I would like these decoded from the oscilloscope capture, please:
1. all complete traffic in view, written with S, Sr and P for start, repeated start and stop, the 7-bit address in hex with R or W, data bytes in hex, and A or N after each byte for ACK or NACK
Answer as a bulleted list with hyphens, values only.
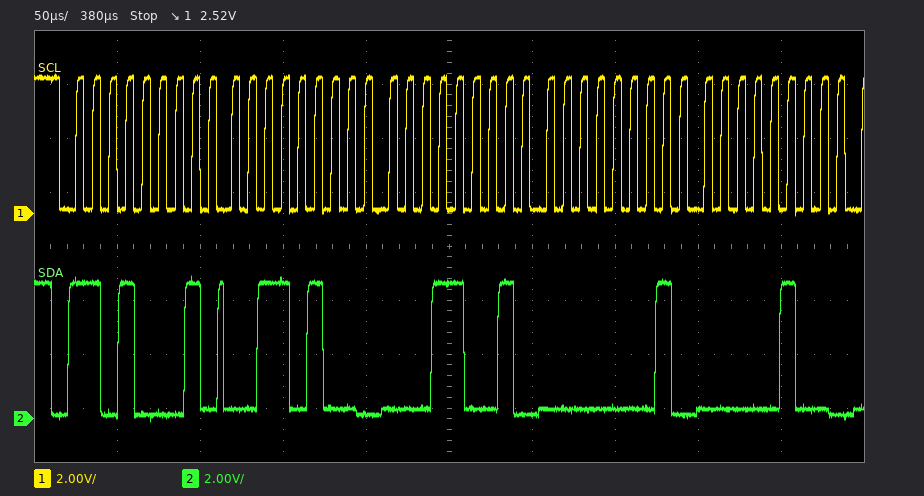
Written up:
- S 68R A 34 A 19 A 01 A 04 A
